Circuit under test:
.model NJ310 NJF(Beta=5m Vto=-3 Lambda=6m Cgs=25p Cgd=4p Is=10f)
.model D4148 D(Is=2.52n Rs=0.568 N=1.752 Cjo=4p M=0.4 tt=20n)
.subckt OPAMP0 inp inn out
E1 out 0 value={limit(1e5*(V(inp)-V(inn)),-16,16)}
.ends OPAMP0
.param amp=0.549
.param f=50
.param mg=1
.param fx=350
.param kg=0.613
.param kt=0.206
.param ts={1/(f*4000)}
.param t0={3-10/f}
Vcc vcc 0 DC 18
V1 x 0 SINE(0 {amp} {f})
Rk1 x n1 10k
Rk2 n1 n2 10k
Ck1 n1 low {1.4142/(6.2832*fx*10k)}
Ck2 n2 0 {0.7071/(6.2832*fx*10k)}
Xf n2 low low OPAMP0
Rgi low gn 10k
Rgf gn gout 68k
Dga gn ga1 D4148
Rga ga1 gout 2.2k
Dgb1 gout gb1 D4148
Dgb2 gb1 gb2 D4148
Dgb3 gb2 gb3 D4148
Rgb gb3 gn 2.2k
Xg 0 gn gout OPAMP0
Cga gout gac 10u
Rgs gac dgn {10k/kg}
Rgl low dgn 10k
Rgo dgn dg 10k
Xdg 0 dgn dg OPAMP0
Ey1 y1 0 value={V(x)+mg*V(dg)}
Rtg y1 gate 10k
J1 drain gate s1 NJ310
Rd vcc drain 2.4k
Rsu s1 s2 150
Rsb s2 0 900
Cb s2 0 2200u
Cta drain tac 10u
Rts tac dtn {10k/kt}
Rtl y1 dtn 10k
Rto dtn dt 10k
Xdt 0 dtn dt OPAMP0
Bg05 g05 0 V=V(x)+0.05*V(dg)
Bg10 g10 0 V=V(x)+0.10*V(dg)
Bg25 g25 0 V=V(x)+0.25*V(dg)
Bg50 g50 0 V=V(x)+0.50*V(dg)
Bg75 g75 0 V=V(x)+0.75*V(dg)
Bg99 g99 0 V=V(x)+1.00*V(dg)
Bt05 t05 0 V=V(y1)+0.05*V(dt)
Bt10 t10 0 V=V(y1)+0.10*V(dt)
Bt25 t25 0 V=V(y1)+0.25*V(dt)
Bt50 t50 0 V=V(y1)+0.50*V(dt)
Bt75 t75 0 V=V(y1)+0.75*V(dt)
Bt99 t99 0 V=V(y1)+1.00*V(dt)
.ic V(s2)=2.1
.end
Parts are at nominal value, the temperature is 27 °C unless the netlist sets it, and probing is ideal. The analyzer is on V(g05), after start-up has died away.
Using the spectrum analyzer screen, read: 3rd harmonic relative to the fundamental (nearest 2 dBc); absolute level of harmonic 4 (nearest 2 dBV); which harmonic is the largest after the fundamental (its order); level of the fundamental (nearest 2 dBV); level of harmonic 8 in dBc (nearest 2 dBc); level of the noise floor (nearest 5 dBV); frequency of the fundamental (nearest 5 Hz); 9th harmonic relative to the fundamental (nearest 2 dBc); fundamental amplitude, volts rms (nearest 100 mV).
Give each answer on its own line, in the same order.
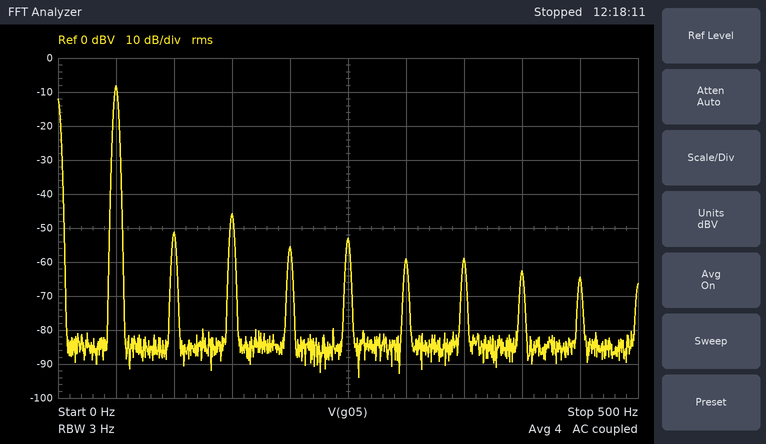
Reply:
-38 dBc
-56 dBV
3
-8 dBV
-54 dBc
-85 dBV
50 Hz
-56 dBc
400 mV
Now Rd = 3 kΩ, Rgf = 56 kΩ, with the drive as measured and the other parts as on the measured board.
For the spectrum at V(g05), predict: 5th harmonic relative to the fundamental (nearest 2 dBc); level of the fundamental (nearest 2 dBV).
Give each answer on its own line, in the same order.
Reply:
-46 dBc
-8 dBV
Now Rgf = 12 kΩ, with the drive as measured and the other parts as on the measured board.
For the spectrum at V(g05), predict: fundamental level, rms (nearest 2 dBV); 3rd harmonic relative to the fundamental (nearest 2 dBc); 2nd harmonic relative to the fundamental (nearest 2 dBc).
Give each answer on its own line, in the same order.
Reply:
-8 dBV
-56 dBc
-50 dBc
